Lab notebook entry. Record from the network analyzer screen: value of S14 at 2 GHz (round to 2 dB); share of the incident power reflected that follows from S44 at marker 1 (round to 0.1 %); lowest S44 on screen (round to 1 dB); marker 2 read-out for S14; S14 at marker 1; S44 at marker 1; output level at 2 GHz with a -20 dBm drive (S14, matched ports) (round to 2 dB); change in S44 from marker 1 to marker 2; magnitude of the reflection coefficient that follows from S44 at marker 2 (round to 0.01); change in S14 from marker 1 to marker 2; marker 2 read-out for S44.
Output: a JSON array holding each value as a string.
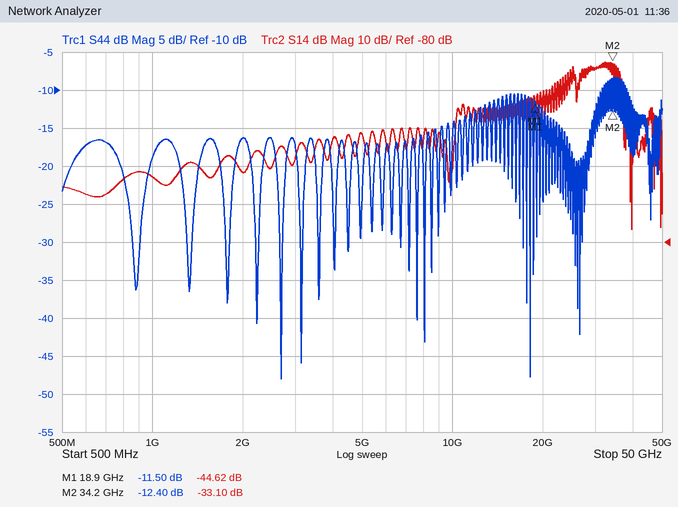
["-62 dB", "7.1 %", "-48 dB", "-33.10 dB", "-44.62 dB", "-11.50 dB", "-82 dBm", "-0.90 dB", "0.24", "11.52 dB", "-12.40 dB"]
